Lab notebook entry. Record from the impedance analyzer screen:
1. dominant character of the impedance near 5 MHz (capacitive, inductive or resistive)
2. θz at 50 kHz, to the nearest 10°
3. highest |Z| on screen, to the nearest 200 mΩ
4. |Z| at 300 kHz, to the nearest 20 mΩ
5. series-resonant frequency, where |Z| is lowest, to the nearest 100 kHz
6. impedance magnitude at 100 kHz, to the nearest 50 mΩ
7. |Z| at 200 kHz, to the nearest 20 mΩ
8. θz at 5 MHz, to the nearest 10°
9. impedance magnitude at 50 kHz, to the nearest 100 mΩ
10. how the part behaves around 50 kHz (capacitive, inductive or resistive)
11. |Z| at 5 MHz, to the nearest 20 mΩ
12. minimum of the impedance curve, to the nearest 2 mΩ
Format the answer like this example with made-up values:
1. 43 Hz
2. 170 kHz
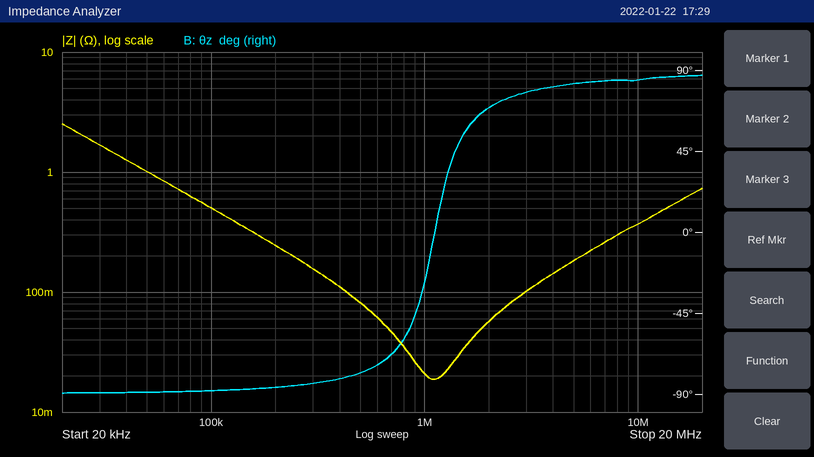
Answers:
1. inductive
2. -90°
3. 2.6 Ω
4. 160 mΩ
5. 1.1 MHz
6. 500 mΩ
7. 240 mΩ
8. 80°
9. 1.0 Ω
10. capacitive
11. 180 mΩ
12. 18 mΩ
